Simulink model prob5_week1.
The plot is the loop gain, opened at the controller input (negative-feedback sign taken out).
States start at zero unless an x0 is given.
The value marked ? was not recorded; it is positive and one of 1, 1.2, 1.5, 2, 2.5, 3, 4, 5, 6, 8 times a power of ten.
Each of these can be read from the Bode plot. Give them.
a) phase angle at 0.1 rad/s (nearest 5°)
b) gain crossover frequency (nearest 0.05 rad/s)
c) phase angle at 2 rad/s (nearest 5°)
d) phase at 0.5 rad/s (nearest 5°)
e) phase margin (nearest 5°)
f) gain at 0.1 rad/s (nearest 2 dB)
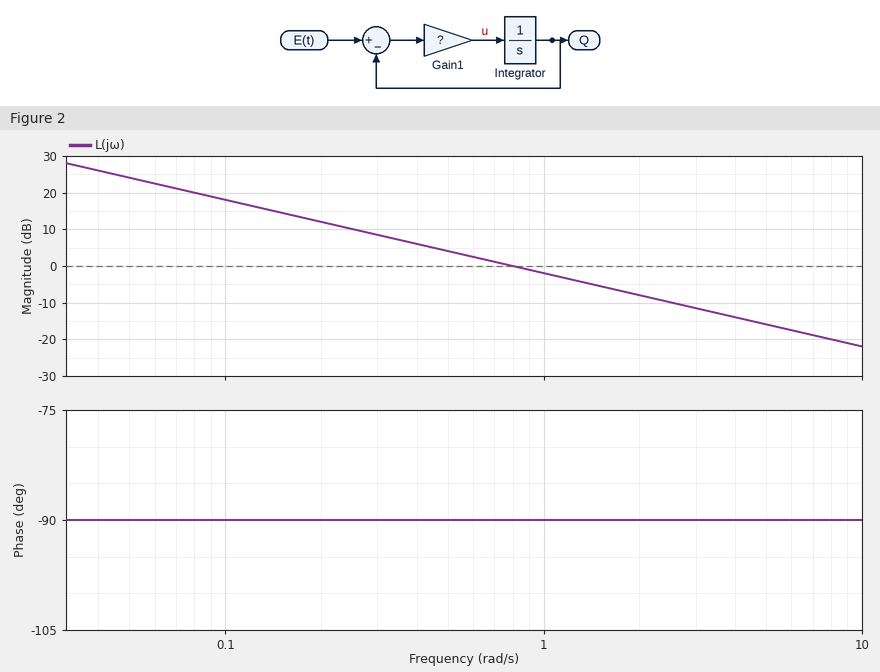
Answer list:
-90°
0.80 rad/s
-90°
-90°
90°
18 dB
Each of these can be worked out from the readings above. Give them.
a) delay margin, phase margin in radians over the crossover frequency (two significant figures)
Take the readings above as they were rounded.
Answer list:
2.0 s
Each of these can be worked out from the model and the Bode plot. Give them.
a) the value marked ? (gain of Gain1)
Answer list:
0.8
